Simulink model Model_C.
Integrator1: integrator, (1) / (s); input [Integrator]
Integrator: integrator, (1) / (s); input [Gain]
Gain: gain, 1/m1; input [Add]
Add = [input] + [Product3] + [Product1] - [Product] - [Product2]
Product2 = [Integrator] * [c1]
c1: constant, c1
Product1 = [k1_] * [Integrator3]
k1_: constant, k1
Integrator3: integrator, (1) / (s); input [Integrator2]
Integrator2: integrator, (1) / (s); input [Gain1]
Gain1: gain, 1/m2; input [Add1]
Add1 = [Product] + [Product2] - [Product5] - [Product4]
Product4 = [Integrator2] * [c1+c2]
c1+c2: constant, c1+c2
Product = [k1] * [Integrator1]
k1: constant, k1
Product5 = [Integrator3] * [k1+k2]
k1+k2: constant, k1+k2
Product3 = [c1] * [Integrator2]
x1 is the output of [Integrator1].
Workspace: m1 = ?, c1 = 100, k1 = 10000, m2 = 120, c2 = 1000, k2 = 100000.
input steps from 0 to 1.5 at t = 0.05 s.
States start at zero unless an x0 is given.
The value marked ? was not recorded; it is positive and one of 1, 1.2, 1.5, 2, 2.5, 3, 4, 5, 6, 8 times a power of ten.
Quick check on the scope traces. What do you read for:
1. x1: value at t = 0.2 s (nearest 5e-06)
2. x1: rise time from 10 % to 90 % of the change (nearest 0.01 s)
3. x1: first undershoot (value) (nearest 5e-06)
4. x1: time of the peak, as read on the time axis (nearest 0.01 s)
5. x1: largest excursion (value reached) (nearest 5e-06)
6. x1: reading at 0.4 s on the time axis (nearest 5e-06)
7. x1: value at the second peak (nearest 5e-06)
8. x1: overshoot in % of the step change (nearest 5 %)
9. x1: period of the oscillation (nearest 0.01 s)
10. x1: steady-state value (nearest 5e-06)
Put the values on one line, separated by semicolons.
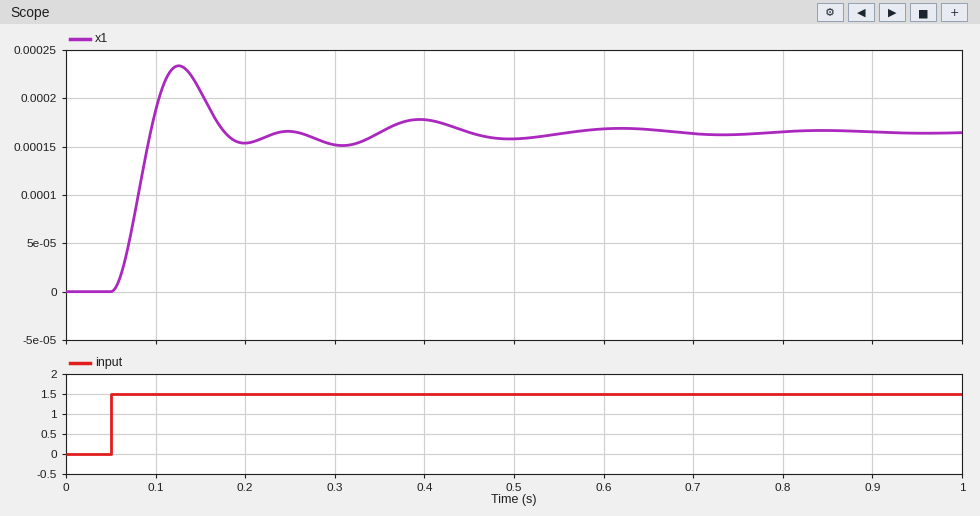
0.000155; 0.03 s; 0.000150; 0.13 s; 0.000235; 0.000180; 0.000180; 40 %; 0.27 s; 0.000165
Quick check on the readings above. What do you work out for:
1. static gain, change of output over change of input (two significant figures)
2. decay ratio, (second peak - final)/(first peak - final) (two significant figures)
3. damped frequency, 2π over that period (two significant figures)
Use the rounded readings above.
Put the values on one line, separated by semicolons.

0.00011; 0.21; 23 rad/s
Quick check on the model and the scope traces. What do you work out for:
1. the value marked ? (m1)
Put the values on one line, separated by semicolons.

5
